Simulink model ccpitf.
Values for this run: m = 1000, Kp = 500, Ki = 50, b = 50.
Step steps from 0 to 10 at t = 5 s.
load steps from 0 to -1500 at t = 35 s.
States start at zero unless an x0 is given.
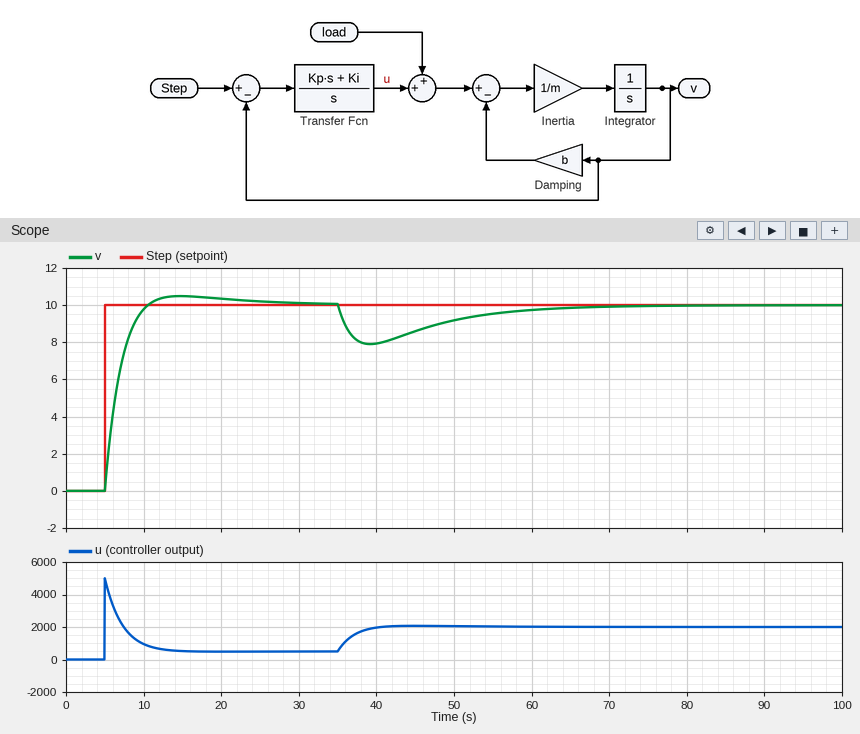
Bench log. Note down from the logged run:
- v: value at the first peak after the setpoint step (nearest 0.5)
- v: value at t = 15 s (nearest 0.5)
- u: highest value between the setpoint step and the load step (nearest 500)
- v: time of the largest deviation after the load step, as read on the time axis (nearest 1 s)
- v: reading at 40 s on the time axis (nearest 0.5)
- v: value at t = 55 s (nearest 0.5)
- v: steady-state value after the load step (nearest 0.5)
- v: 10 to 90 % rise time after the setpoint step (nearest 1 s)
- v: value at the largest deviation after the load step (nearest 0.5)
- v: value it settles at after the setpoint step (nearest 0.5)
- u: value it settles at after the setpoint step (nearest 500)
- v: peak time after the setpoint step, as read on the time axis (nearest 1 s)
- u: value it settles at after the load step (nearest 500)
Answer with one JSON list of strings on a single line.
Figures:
["10.5", "10.5", "5000", "39 s", "8.0", "9.5", "10.0", "4 s", "8.0", "10.0", "500", "15 s", "2000"]
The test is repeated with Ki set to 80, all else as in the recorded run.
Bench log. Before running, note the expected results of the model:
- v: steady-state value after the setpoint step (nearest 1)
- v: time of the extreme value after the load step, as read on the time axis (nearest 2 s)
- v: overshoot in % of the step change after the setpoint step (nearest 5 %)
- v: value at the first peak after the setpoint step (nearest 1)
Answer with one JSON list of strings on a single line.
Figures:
["10", "38 s", "10 %", "11"]
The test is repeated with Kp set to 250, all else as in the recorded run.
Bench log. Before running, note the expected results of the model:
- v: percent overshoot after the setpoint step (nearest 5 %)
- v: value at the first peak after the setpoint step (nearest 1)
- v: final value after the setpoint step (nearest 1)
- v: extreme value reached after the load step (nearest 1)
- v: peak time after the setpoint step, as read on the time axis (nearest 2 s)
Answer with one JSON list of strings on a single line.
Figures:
["15 %", "12", "10", "7", "16 s"]
